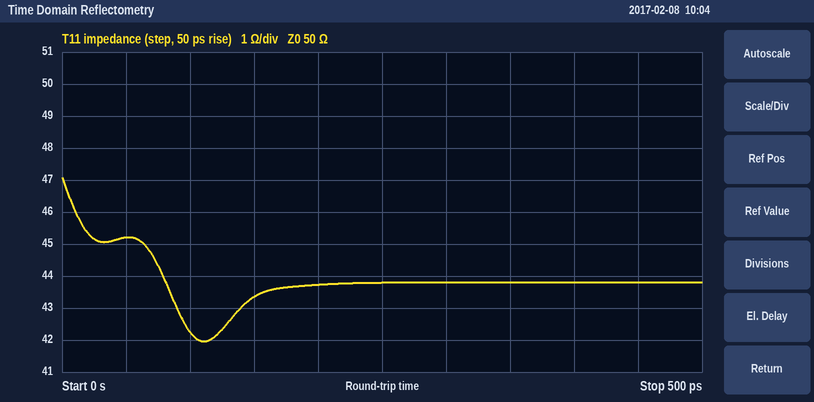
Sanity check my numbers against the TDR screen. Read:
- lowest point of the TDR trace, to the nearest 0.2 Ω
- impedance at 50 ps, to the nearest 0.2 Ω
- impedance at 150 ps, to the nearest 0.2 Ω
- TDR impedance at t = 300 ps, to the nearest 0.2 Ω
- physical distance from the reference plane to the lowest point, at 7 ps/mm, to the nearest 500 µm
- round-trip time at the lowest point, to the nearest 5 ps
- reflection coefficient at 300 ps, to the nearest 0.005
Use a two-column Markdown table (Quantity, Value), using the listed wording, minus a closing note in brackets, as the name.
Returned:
| Quantity | Value |
|---|---|
| lowest point of the TDR trace, to the nearest 0.2 Ω | 42.0 Ω |
| impedance at 50 ps, to the nearest 0.2 Ω | 45.2 Ω |
| impedance at 150 ps, to the nearest 0.2 Ω | 43.4 Ω |
| TDR impedance at t = 300 ps, to the nearest 0.2 Ω | 43.8 Ω |
| physical distance from the reference plane to the lowest point, at 7 ps/mm, to the nearest 500 µm | 8.0 mm |
| round-trip time at the lowest point, to the nearest 5 ps | 110 ps |
| reflection coefficient at 300 ps, to the nearest 0.005 | -0.065 |
